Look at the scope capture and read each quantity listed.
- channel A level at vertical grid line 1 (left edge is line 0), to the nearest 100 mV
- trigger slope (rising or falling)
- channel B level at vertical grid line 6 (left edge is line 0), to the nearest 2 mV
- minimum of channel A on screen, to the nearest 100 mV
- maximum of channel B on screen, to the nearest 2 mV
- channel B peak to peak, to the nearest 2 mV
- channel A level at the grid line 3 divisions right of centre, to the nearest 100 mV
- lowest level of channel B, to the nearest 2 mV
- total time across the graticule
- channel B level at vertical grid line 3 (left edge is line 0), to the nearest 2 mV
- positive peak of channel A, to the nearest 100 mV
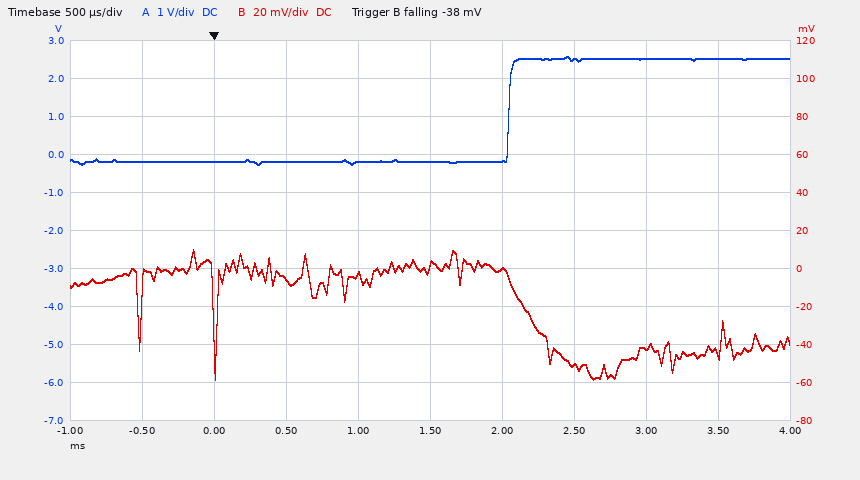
-200 mV
falling
0 mV
-300 mV
10 mV
68 mV
2.5 V
-58 mV
5 ms
-6 mV
2.6 V
